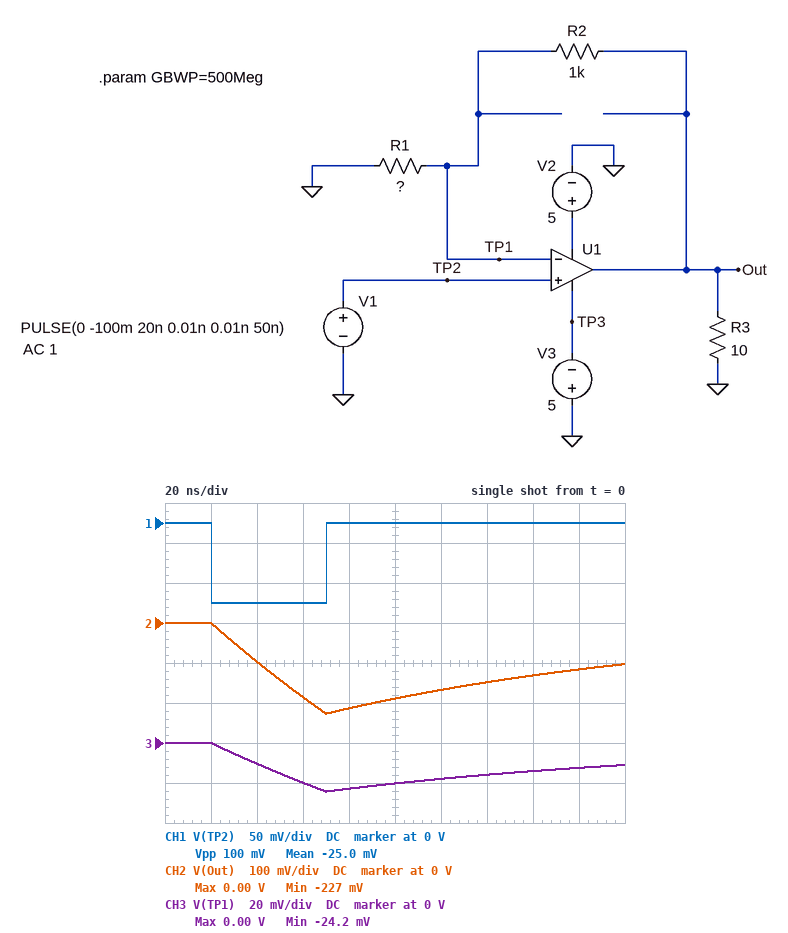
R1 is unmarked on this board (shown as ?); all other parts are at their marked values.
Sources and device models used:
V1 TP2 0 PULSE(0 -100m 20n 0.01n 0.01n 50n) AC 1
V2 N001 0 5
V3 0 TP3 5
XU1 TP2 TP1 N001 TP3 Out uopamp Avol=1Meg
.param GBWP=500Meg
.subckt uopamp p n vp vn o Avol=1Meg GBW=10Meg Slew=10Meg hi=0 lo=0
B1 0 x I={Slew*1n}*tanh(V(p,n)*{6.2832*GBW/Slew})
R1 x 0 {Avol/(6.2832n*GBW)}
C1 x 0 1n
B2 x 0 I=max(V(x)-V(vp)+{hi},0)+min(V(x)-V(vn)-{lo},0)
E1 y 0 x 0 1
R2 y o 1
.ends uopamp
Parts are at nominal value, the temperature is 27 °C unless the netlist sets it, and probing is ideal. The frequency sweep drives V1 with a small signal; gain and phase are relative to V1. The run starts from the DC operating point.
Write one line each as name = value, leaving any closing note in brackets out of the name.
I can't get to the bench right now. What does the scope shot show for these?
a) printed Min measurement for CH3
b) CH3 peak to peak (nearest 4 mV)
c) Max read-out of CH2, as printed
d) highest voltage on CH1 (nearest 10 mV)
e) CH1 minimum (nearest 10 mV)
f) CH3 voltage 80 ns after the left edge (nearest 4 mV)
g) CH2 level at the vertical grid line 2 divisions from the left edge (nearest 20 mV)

printed Min measurement for CH3 = -24.2 mV
CH3 peak to peak = 24 mV
Max read-out of CH2, as printed = 0.00 V
highest voltage on CH1 = 0 V
CH1 minimum = -100 mV
CH3 voltage 80 ns after the left edge = -24 mV
CH2 level at the vertical grid line 2 divisions from the left edge = -100 mV
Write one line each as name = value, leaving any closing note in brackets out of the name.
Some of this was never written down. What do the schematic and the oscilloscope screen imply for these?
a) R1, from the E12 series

R1, from the E12 series = 120 Ω
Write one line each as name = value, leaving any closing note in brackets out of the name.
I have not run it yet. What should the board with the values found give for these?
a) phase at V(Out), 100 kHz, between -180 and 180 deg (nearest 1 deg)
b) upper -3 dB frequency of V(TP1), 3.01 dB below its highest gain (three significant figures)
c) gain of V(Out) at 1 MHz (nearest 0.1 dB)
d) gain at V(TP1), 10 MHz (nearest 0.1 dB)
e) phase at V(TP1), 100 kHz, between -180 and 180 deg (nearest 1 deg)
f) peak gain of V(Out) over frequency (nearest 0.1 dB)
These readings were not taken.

phase at V(Out), 100 kHz, between -180 and 180 deg = -6 deg
upper -3 dB frequency of V(TP1), 3.01 dB below its highest gain = 973 kHz
gain of V(Out) at 1 MHz = 16.3 dB
gain at V(TP1), 10 MHz = -20.3 dB
phase at V(TP1), 100 kHz, between -180 and 180 deg = -6 deg
peak gain of V(Out) over frequency = 19.4 dB
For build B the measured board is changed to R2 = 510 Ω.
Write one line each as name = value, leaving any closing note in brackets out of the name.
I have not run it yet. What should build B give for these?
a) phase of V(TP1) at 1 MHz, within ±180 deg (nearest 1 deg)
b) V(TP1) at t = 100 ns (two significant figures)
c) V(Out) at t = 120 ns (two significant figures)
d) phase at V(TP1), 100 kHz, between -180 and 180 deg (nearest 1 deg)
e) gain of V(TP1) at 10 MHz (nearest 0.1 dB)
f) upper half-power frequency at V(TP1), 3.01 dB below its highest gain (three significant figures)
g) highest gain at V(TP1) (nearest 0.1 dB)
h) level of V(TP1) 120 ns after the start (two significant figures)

phase of V(TP1) at 1 MHz, within ±180 deg = -30 deg
V(TP1) at t = 100 ns = -29 mV
V(Out) at t = 120 ns = -120 mV
phase at V(TP1), 100 kHz, between -180 and 180 deg = -3 deg
gain of V(TP1) at 10 MHz = -15.4 dB
upper half-power frequency at V(TP1), 3.01 dB below its highest gain = 1.73 MHz
highest gain at V(TP1) = 0 dB
level of V(TP1) 120 ns after the start = -23 mV
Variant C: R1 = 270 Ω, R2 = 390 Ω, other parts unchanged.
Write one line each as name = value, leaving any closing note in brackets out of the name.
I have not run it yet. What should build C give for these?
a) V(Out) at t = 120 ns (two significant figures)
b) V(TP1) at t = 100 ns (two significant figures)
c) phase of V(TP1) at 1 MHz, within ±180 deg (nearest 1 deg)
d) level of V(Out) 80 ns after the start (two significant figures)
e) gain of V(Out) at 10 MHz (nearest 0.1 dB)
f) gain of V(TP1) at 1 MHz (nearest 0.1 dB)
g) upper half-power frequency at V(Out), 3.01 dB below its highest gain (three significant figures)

V(Out) at t = 120 ns = -52 mV
V(TP1) at t = 100 ns = -34 mV
phase of V(TP1) at 1 MHz, within ±180 deg = -15 deg
level of V(Out) 80 ns after the start = -130 mV
gain of V(Out) at 10 MHz = -1.4 dB
gain of V(TP1) at 1 MHz = -0.3 dB
upper half-power frequency at V(Out), 3.01 dB below its highest gain = 3.71 MHz
